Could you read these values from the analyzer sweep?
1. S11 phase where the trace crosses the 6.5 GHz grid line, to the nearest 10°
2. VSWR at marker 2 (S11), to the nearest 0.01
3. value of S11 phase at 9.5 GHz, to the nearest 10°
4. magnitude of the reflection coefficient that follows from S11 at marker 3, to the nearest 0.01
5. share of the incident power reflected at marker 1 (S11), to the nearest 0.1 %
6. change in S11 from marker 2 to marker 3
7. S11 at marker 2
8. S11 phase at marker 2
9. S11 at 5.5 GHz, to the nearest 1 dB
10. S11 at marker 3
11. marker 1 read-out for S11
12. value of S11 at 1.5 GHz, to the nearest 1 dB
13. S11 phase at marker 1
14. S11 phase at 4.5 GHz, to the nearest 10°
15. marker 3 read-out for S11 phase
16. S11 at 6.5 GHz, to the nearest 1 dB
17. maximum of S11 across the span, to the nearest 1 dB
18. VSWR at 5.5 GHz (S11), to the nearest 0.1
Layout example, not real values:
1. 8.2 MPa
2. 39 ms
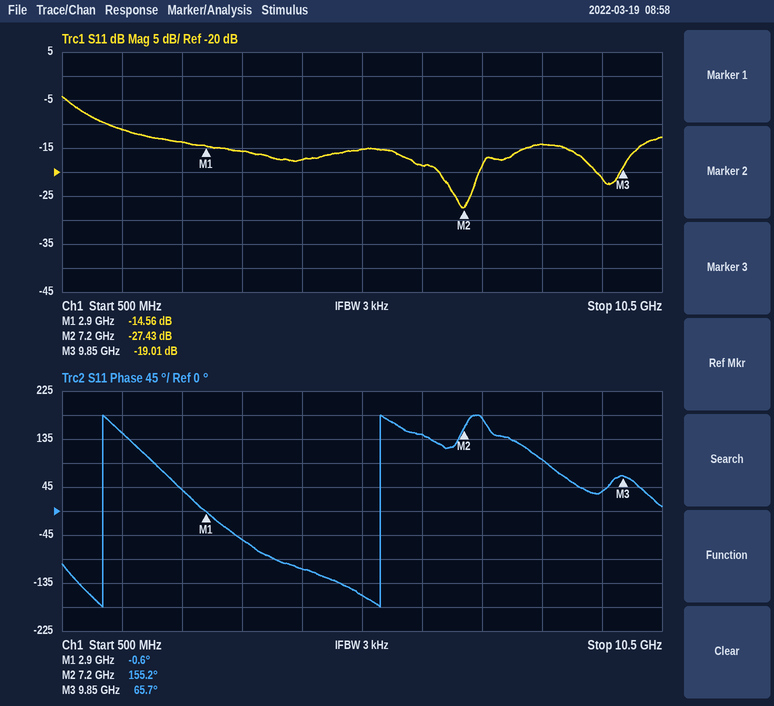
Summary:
1. 140°
2. 1.09
3. 40°
4. 0.11
5. 3.5 %
6. 8.42 dB
7. -27.43 dB
8. 155.2°
9. -15 dB
10. -19.01 dB
11. -14.56 dB
12. -11 dB
13. -0.6°
14. -110°
15. 65.7°
16. -19 dB
17. -4 dB
18. 1.4
